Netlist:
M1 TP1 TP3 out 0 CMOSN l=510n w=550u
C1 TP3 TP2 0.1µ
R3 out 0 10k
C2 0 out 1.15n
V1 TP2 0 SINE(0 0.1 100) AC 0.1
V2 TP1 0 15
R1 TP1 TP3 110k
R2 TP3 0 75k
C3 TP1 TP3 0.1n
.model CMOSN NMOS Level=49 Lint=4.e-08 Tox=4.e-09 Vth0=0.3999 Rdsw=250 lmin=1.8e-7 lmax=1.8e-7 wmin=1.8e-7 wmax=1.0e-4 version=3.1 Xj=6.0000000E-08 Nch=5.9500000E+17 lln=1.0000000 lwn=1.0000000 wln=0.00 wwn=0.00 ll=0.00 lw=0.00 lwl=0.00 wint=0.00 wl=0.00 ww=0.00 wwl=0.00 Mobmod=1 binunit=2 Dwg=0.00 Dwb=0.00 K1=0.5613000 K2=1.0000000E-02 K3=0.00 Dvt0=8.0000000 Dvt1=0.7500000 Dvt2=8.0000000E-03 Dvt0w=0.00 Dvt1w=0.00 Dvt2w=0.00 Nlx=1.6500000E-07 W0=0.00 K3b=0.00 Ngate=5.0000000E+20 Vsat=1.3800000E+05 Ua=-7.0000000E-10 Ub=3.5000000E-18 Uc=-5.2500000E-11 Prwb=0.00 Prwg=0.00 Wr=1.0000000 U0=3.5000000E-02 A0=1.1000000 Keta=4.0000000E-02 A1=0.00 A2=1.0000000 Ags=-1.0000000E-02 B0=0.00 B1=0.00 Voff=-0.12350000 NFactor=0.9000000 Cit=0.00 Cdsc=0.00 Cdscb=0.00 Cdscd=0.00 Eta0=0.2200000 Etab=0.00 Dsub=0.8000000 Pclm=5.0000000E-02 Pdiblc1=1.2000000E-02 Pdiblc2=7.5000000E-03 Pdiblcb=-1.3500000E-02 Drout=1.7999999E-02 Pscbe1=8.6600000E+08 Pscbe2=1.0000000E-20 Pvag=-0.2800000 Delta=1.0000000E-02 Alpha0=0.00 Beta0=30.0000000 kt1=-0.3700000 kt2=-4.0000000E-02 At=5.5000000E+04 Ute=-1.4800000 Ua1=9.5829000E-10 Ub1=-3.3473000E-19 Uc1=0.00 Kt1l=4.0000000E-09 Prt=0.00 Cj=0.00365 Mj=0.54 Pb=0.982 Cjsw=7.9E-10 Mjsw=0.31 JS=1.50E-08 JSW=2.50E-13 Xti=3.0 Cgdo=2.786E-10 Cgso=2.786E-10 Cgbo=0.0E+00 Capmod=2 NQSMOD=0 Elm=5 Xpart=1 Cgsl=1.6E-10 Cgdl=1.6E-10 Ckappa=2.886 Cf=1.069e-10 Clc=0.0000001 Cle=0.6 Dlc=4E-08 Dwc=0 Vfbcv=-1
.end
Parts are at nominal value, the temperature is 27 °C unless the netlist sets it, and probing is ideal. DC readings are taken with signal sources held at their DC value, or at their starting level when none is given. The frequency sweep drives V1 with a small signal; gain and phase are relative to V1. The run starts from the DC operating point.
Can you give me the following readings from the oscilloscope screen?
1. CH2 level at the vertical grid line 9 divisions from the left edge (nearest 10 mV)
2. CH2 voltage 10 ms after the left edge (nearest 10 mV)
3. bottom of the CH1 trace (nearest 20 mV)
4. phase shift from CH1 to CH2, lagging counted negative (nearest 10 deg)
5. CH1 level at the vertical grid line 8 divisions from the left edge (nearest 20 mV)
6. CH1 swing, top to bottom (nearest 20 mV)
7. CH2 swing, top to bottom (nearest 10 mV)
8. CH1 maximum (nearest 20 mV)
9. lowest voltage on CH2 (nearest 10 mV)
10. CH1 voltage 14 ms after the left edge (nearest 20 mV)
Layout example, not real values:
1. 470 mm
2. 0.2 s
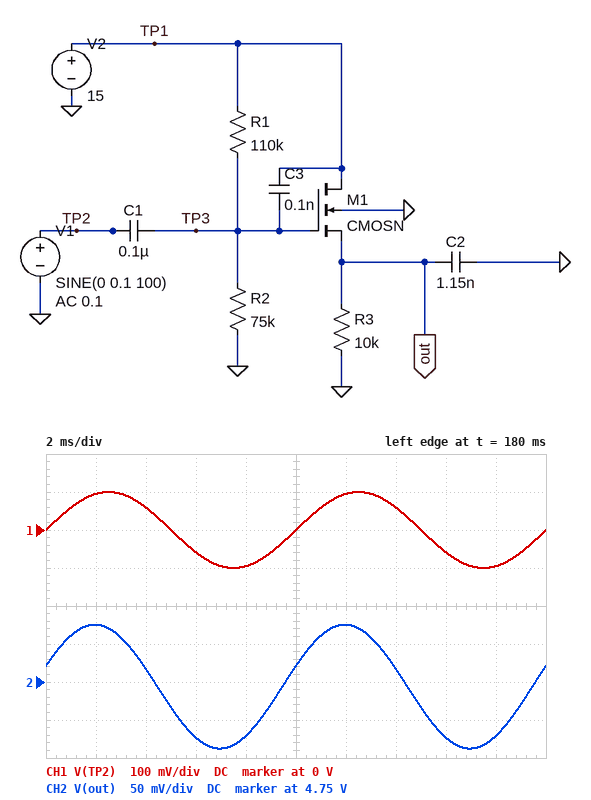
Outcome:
1. 4.68 V
2. 4.77 V
3. -100 mV
4. 20 deg
5. -60 mV
6. 200 mV
7. 160 mV
8. 100 mV
9. 4.66 V
10. 60 mV
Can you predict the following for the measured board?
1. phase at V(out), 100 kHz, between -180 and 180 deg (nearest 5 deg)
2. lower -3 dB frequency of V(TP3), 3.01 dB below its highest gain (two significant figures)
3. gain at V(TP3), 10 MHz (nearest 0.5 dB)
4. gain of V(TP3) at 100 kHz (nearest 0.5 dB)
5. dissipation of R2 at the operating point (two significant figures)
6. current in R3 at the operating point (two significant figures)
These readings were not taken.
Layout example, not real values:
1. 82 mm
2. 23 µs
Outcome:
1. -5 deg
2. 36 Hz
3. 0 dB
4. 0 dB
5. 490 µW
6. 470 µA
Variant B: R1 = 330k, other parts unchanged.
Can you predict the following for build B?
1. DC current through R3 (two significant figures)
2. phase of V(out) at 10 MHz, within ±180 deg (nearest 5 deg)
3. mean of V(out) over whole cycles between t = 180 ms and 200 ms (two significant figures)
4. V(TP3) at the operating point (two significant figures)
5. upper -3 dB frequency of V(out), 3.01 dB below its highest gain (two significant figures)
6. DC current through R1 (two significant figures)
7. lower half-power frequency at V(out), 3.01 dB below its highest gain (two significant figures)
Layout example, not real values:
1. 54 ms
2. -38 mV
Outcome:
1. 190 µA
2. -85 deg
3. 1.9 V
4. 2.8 V
5. 760 kHz
6. 37 µA
7. 26 Hz
